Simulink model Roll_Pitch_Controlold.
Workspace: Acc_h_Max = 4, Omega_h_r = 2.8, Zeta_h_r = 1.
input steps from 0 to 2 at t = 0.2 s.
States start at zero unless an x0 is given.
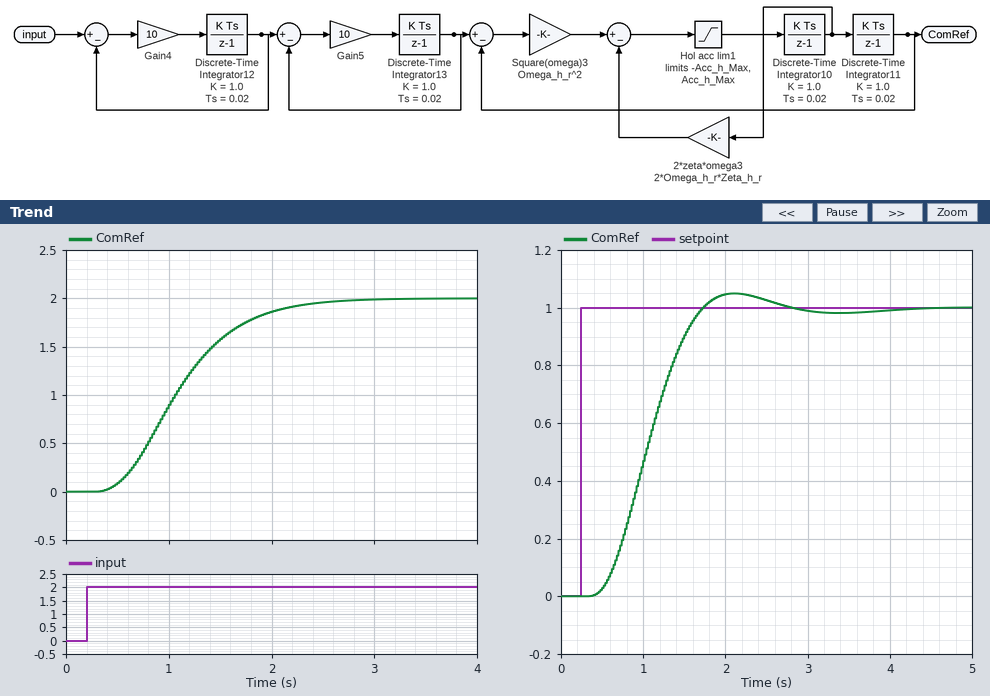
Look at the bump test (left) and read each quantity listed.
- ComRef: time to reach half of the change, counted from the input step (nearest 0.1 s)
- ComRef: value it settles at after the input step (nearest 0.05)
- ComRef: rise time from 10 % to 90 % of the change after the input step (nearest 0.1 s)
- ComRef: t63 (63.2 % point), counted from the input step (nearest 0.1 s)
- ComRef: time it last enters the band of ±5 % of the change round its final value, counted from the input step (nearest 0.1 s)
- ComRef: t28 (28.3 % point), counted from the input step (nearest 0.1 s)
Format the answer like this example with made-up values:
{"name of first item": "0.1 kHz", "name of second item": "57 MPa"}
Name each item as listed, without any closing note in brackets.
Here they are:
{"ComRef: time to reach half of the change, counted from the input step": "0.9 s", "ComRef: value it settles at after the input step": "2.00", "ComRef: rise time from 10 % to 90 % of the change after the input step": "1.2 s", "ComRef: t63 (63.2 % point), counted from the input step": "1.0 s", "ComRef: time it last enters the band of ±5 % of the change round its final value, counted from the input step": "1.9 s", "ComRef: t28 (28.3 % point), counted from the input step": "0.6 s"}
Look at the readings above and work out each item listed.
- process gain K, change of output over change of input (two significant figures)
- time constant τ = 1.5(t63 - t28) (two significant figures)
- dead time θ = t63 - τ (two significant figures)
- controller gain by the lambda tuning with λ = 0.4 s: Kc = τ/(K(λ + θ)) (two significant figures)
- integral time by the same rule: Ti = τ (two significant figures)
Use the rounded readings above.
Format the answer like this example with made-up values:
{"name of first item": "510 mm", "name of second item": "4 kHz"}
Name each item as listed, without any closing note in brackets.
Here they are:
{"process gain K, change of output over change of input": "1.0", "time constant τ = 1.5(t63 - t28)": "0.60 s", "dead time θ = t63 - τ": "0.40 s", "controller gain by the lambda tuning with λ = 0.4 s: Kc = τ/(K(λ + θ))": "0.75", "integral time by the same rule: Ti = τ": "0.60 s"}
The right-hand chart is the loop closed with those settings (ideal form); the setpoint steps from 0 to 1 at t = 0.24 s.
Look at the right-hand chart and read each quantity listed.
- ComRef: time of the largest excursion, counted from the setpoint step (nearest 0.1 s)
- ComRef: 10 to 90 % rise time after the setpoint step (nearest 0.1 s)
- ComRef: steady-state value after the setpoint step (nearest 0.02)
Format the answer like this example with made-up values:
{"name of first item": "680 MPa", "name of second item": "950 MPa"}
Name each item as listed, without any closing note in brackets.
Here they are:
{"ComRef: time of the largest excursion, counted from the setpoint step": "1.9 s", "ComRef: 10 to 90 % rise time after the setpoint step": "0.9 s", "ComRef: steady-state value after the setpoint step": "1.00"}
